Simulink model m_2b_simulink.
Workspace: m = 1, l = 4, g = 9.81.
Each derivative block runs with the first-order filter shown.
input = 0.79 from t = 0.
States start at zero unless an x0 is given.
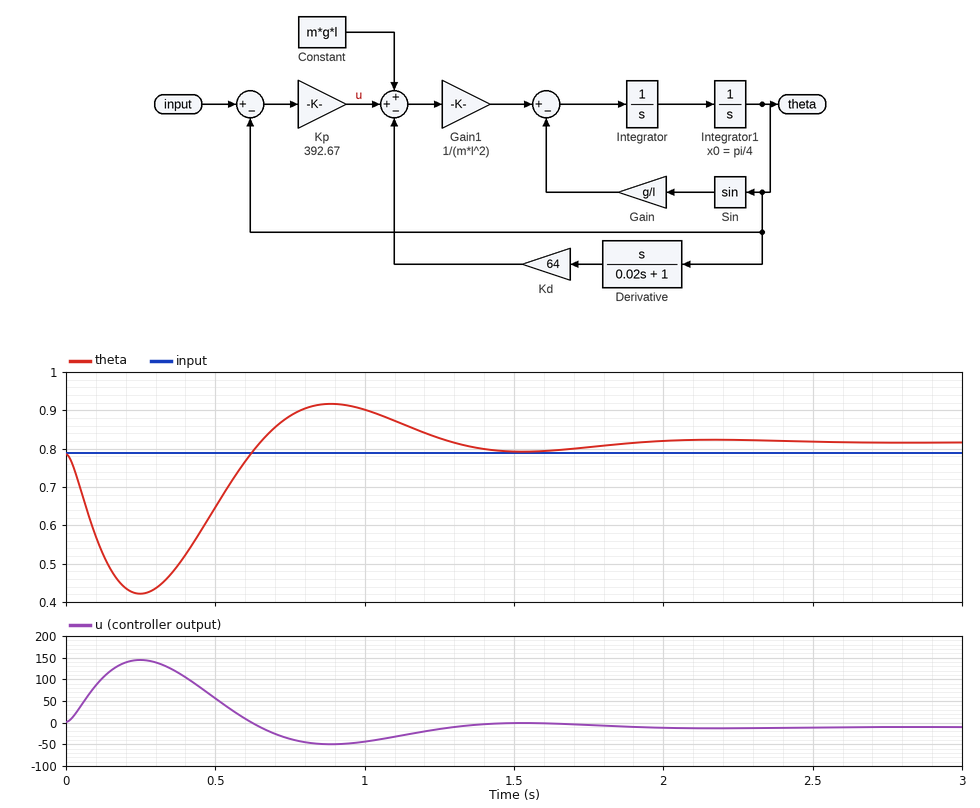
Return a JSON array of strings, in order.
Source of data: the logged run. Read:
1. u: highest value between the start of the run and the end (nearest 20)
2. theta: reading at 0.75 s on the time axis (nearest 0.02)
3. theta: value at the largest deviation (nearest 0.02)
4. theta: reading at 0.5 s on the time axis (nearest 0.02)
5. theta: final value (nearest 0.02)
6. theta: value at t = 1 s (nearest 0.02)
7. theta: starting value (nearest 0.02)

["140", "0.88", "0.42", "0.64", "0.82", "0.90", "0.78"]
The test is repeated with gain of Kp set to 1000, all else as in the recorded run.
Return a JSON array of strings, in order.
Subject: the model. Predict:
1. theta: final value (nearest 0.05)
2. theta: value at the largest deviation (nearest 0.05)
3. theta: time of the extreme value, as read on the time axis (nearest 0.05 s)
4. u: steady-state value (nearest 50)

["0.80", "0.50", "0.20 s", "0"]
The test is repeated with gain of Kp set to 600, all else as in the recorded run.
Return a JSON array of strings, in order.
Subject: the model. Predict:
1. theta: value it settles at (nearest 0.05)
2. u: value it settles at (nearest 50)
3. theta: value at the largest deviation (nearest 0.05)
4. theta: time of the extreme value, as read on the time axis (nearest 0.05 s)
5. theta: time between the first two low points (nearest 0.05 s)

["0.80", "0", "0.45", "0.20 s", "1.00 s"]
